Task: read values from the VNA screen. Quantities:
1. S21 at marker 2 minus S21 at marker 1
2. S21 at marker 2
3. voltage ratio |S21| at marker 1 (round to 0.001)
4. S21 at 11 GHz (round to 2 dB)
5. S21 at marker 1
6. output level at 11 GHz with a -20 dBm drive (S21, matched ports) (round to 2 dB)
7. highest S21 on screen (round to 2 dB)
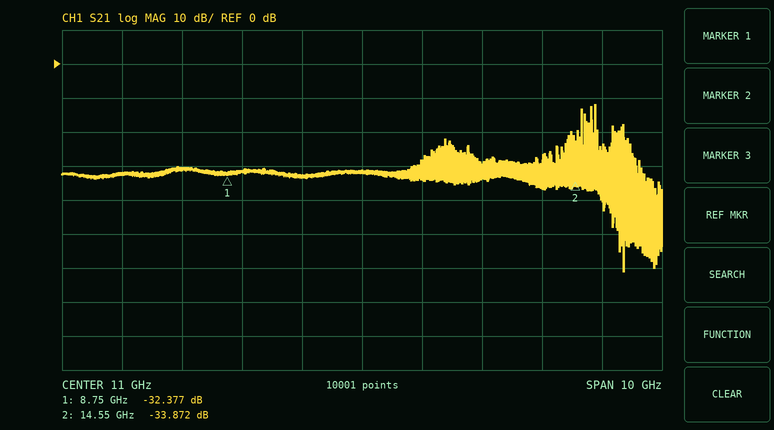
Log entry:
-1.495 dB
-33.872 dB
0.024
-32 dB
-32.377 dB
-52 dBm
-12 dB
